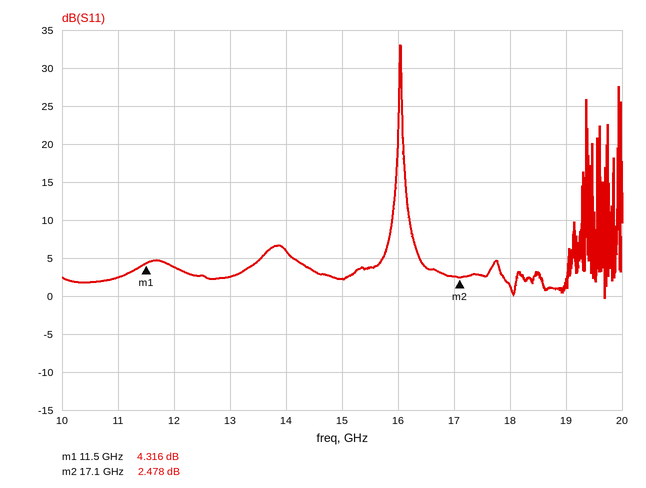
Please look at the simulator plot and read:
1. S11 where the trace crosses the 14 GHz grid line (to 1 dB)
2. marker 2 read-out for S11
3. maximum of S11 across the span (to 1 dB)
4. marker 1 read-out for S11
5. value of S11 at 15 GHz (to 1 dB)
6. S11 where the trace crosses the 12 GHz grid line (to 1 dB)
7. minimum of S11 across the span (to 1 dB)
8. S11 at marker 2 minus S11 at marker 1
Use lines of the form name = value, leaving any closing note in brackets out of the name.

S11 where the trace crosses the 14 GHz grid line = 6 dB
marker 2 read-out for S11 = 2.478 dB
maximum of S11 across the span = 33 dB
marker 1 read-out for S11 = 4.316 dB
value of S11 at 15 GHz = 2 dB
S11 where the trace crosses the 12 GHz grid line = 4 dB
minimum of S11 across the span = 0 dB
S11 at marker 2 minus S11 at marker 1 = -1.838 dB
